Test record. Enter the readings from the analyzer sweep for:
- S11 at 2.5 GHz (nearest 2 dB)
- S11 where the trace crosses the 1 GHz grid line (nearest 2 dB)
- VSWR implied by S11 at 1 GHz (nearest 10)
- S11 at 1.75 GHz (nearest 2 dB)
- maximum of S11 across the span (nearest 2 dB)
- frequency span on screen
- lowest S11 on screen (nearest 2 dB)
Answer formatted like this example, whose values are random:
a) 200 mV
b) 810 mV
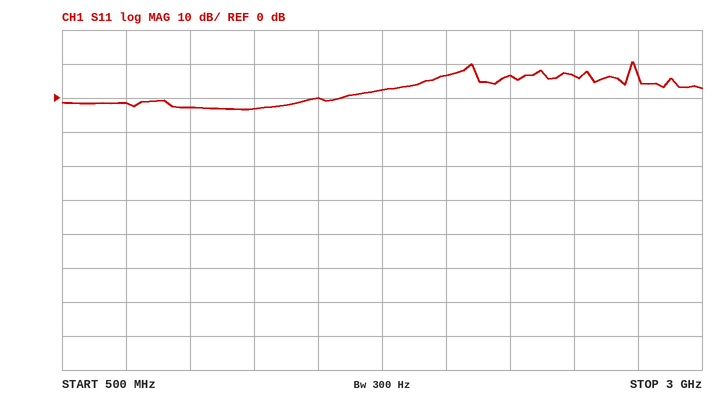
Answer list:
a) 6 dB
b) -2 dB
c) 10
d) 2 dB
e) 10 dB
f) 2.5 GHz
g) -4 dB
